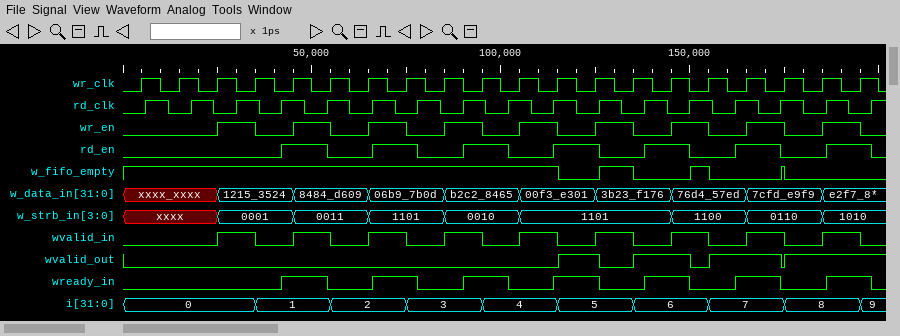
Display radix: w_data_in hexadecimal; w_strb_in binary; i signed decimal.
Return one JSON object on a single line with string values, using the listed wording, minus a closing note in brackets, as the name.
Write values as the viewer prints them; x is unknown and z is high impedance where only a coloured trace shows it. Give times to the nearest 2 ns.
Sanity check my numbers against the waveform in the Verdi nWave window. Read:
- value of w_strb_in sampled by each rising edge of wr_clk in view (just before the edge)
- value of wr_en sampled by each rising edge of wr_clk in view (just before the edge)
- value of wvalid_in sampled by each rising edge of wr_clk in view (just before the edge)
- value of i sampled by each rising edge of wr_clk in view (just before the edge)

{"value of w_strb_in sampled by each rising edge of wr_clk in view": "xxxx, xxxx, xxxx, 0001, 0001, 0011, 0011, 1101, 1101, 0010, 0010, 1101, 1101, 1101, 1101, 1100, 1100, 0110, 0110, 1010", "value of wr_en sampled by each rising edge of wr_clk in view": "0 0 0 1 0 1 0 1 0 1 0 1 0 1 0 1 0 1 0 1", "value of wvalid_in sampled by each rising edge of wr_clk in view": "0 0 0 1 0 1 0 1 0 1 0 1 0 1 0 1 0 1 0 1", "value of i sampled by each rising edge of wr_clk in view": "0, 0, 0, 0, 1, 1, 2, 2, 3, 3, 4, 4, 5, 5, 6, 6, 7, 7, 8, 8"}
